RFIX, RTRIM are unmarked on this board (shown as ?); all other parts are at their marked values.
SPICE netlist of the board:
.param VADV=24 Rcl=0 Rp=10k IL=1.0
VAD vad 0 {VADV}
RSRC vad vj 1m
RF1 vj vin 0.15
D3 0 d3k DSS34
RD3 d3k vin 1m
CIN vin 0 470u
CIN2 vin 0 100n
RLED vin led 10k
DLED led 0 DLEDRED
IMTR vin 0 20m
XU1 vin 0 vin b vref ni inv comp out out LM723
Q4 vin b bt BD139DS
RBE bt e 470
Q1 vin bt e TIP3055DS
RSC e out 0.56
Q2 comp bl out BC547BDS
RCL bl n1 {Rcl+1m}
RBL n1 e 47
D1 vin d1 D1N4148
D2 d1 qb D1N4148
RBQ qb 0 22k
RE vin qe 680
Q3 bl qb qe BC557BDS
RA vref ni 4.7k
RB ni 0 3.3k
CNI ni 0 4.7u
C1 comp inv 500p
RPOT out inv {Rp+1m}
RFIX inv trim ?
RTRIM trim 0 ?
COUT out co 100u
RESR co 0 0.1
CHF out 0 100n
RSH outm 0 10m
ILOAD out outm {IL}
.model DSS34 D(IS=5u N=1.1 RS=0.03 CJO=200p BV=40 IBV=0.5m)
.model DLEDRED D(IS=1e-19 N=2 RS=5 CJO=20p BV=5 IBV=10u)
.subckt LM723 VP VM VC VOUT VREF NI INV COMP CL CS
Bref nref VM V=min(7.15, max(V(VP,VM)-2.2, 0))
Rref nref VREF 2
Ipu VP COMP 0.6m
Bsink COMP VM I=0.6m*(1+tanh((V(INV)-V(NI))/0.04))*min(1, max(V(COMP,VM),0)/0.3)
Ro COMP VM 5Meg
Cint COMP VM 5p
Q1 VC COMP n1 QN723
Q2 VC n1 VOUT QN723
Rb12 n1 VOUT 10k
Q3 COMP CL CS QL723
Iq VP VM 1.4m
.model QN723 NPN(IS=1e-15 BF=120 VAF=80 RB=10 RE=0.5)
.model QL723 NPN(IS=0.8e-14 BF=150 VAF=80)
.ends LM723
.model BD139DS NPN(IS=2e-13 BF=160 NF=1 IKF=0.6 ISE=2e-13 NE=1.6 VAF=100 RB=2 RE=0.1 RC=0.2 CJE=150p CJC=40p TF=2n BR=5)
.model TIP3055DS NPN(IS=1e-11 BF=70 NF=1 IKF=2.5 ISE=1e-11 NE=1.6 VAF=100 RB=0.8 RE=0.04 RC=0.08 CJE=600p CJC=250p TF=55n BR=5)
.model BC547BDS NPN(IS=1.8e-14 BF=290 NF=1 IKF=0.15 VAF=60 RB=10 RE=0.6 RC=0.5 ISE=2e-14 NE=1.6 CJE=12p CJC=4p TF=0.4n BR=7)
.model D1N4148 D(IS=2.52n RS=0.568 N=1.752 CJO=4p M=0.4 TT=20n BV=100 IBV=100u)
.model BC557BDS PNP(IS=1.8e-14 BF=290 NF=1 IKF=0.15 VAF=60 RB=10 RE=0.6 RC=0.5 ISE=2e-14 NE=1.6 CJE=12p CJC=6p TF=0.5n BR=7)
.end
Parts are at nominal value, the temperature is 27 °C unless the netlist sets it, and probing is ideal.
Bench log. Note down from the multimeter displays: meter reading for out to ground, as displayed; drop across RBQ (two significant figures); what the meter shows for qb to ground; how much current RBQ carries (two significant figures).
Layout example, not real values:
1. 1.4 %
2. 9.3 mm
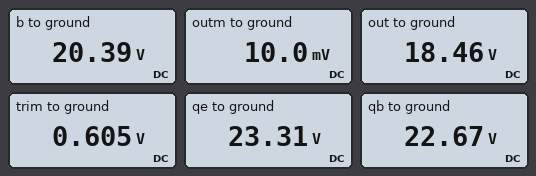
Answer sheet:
1. 18.46 V
2. 23 V
3. 22.67 V
4. 1.0 mA
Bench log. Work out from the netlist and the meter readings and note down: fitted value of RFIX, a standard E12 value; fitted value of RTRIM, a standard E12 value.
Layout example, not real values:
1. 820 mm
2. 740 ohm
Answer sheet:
1. 1.5 kΩ
2. 390 Ω
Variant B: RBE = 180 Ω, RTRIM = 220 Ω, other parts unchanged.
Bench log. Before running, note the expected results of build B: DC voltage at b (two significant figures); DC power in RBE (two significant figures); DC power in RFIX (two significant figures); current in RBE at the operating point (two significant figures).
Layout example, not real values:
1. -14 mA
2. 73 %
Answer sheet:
1. 22 V
2. 2.9 mW
3. 4.4 mW
4. 4.0 mA
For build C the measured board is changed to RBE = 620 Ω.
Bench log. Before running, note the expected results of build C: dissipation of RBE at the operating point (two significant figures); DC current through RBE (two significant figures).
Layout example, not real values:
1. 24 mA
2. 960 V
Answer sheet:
1. 830 µW
2. 1.2 mA
